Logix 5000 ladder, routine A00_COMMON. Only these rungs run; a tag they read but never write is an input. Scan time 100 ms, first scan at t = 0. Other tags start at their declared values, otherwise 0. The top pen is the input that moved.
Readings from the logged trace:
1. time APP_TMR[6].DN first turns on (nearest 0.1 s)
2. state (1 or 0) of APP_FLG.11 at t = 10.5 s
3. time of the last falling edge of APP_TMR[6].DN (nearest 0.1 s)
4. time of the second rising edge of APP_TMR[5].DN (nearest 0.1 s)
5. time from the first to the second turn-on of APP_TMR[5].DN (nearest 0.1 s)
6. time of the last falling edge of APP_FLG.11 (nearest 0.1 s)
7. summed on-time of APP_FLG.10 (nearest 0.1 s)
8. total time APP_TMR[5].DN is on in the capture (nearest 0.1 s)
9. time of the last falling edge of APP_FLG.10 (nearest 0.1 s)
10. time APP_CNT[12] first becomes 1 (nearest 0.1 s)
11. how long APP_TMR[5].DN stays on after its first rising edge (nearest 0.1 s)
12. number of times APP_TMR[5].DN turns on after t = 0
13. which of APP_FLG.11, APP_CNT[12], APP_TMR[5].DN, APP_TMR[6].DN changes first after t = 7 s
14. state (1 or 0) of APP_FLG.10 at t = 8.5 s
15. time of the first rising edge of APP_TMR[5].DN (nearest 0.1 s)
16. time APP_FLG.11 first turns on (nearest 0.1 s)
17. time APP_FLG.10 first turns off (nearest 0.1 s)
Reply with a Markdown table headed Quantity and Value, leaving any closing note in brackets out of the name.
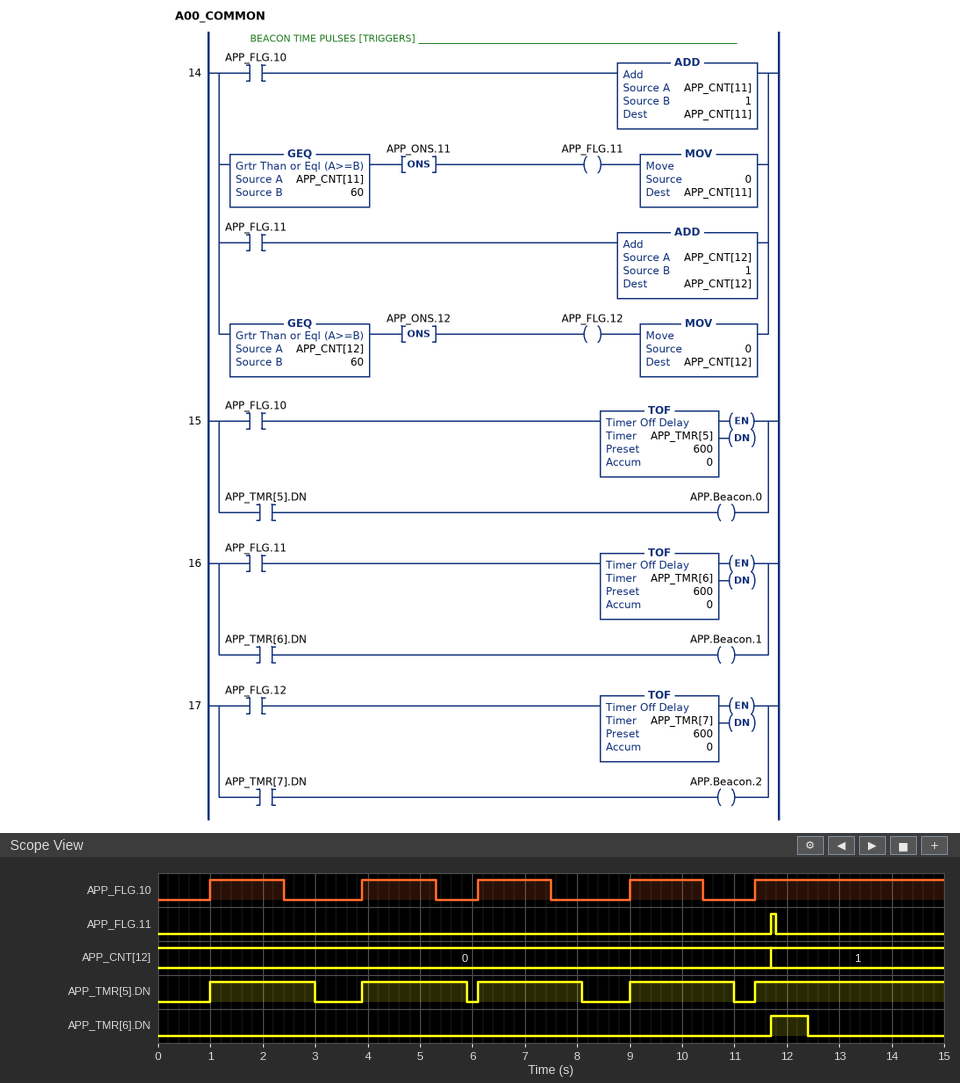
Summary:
| Quantity | Value |
|---|---|
| time APP_TMR[6].DN first turns on | 11.7 s |
| state (1 or 0) of APP_FLG.11 at t = 10.5 s | 0 |
| time of the last falling edge of APP_TMR[6].DN | 12.4 s |
| time of the second rising edge of APP_TMR[5].DN | 3.9 s |
| time from the first to the second turn-on of APP_TMR[5].DN | 2.9 s |
| time of the last falling edge of APP_FLG.11 | 11.8 s |
| summed on-time of APP_FLG.10 | 9.2 s |
| total time APP_TMR[5].DN is on in the capture | 11.6 s |
| time of the last falling edge of APP_FLG.10 | 10.4 s |
| time APP_CNT[12] first becomes 1 | 11.7 s |
| how long APP_TMR[5].DN stays on after its first rising edge | 2.0 s |
| number of times APP_TMR[5].DN turns on after t = 0 | 5 |
| which of APP_FLG.11, APP_CNT[12], APP_TMR[5].DN, APP_TMR[6].DN changes first after t = 7 s | APP_TMR[5].DN |
| state (1 or 0) of APP_FLG.10 at t = 8.5 s | 0 |
| time of the first rising edge of APP_TMR[5].DN | 1.0 s |
| time APP_FLG.11 first turns on | 11.7 s |
| time APP_FLG.10 first turns off | 2.4 s |
